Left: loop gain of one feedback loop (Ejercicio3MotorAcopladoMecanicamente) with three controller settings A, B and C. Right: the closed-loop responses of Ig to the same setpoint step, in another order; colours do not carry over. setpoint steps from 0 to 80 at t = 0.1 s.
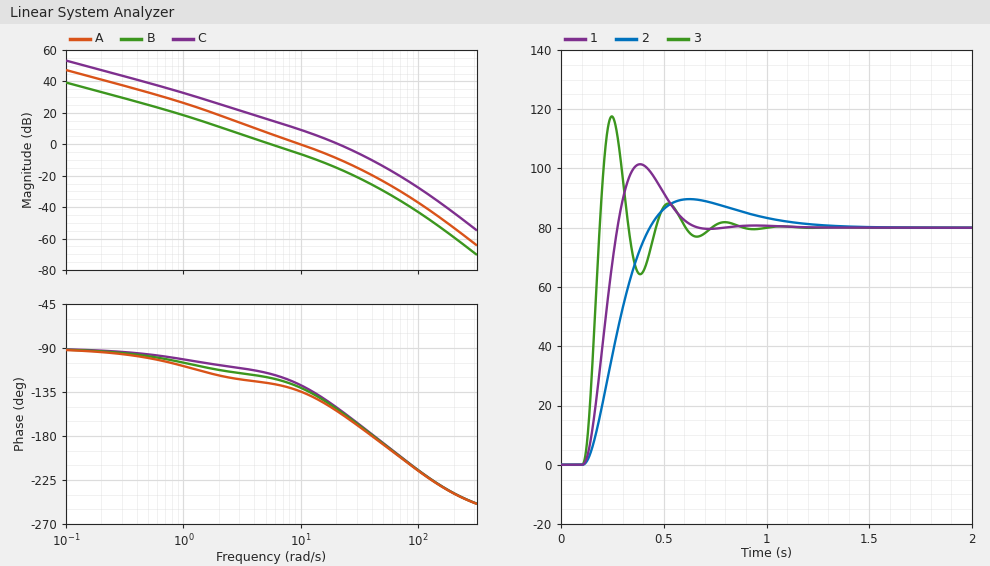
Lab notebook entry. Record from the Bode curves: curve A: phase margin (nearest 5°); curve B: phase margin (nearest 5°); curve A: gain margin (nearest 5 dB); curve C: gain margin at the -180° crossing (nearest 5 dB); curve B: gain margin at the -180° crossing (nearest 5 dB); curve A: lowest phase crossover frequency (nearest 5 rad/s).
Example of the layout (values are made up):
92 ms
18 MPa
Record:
45°
60°
20 dB
10 dB
25 dB
40 rad/s
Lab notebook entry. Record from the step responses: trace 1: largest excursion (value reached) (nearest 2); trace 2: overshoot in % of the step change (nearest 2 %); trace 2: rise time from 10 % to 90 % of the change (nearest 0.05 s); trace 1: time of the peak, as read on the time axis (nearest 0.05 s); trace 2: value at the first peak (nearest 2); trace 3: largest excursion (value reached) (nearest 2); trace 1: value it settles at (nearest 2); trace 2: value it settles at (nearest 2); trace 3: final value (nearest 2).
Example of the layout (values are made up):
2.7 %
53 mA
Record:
102
12 %
0.20 s
0.40 s
90
118
80
80
80
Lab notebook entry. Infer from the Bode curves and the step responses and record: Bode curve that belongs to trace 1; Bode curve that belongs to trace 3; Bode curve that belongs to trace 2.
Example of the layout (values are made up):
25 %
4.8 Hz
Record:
A
C
B
